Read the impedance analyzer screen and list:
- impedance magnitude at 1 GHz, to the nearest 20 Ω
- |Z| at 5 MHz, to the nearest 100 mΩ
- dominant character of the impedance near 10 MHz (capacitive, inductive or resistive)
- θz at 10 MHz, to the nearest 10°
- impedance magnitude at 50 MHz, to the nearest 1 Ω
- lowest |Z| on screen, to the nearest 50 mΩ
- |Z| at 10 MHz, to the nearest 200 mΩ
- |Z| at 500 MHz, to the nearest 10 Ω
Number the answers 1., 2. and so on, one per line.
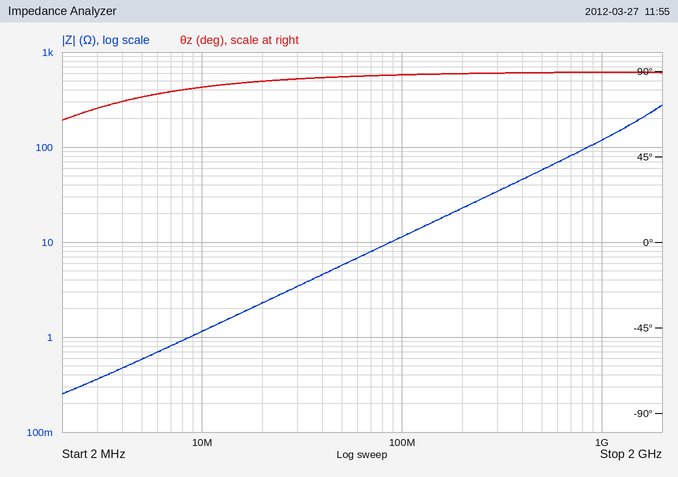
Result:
1. 120 Ω
2. 600 mΩ
3. inductive
4. 80°
5. 6 Ω
6. 250 mΩ
7. 1.2 Ω
8. 60 Ω
